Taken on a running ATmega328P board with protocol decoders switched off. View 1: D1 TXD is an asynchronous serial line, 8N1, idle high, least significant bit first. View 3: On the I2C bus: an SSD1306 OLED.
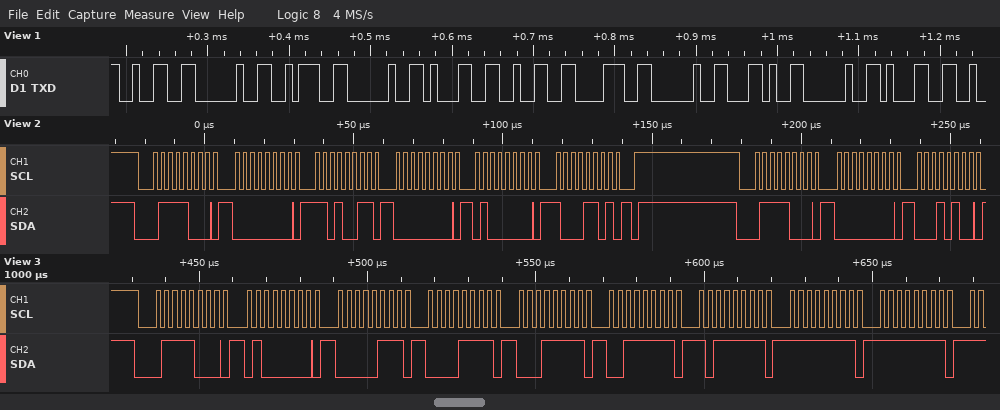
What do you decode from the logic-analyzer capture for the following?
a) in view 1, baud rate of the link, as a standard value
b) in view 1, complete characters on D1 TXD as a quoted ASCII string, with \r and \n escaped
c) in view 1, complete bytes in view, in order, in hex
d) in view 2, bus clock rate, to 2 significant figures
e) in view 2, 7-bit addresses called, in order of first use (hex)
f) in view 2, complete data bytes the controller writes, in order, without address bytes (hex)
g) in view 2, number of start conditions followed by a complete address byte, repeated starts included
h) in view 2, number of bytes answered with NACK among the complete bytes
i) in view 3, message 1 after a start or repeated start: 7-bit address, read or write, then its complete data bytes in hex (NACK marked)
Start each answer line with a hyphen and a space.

- 115200 baud
- "2 : 128 , 1"
- 0x32 0x20 0x3A 0x20 0x31 0x32 0x38 0x20 0x2C 0x20 0x31
- 400 kHz
- 0x3C
- 00 D3 00 40 8D 00 14
- 2
- 0
- 0x3C write: 40 07 0F 1F 3F BF FF FF
